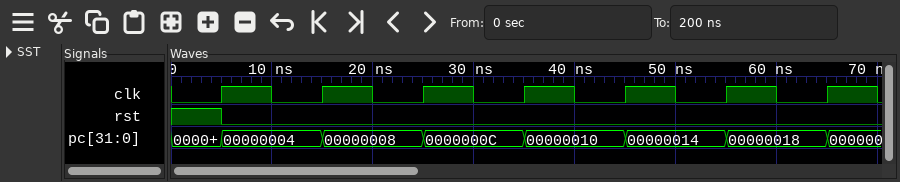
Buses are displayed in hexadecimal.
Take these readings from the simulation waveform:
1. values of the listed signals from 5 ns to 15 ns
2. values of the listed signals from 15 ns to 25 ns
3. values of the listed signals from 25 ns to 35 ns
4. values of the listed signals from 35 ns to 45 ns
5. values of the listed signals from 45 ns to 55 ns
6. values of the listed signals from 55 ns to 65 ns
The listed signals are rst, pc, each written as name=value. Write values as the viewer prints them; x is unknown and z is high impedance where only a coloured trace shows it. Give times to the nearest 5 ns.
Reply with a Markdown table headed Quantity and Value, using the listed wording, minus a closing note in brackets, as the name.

| Quantity | Value |
|---|---|
| values of the listed signals from 5 ns to 15 ns | rst=0, pc=00000004 |
| values of the listed signals from 15 ns to 25 ns | rst=0, pc=00000008 |
| values of the listed signals from 25 ns to 35 ns | rst=0, pc=0000000C |
| values of the listed signals from 35 ns to 45 ns | rst=0, pc=00000010 |
| values of the listed signals from 45 ns to 55 ns | rst=0, pc=00000014 |
| values of the listed signals from 55 ns to 65 ns | rst=0, pc=00000018 |
